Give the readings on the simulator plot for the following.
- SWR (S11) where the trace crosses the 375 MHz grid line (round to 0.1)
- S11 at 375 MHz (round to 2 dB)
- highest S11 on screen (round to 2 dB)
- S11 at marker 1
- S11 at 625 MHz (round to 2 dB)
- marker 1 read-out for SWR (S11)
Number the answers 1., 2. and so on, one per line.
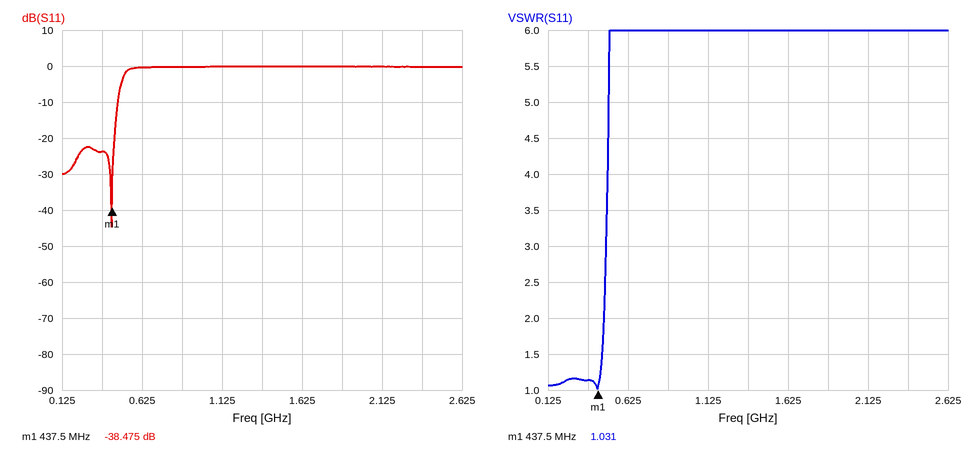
1. 1.1
2. -24 dB
3. 0 dB
4. -38.475 dB
5. 0 dB
6. 1.031
